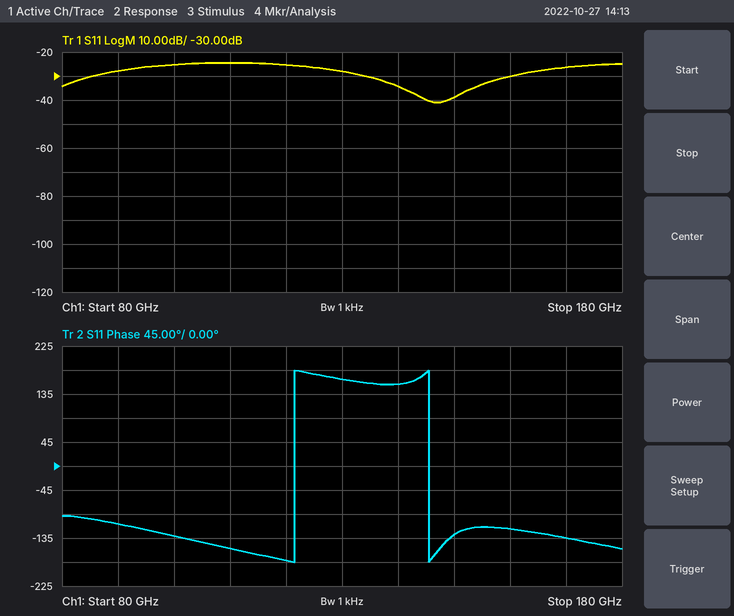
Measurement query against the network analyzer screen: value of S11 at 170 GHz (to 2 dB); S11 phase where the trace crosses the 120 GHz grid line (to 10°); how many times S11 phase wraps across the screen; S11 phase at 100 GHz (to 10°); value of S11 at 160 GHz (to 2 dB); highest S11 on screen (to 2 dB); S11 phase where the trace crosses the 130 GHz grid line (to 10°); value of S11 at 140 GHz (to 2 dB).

-26 dB
-180°
2
-130°
-30 dB
-24 dB
160°
-34 dB
